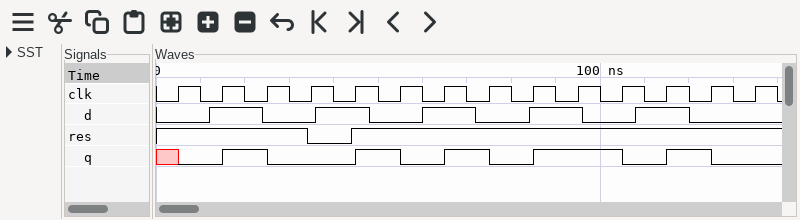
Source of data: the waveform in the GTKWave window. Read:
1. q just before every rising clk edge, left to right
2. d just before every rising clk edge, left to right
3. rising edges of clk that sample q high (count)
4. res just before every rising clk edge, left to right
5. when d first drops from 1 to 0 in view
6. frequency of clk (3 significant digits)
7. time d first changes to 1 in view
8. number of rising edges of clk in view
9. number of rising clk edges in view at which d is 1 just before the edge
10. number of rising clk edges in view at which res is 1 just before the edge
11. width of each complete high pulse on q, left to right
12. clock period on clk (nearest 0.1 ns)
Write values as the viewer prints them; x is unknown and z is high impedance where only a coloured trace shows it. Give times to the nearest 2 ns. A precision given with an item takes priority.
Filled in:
x 0 1 0 0 1 0 1 0 1 1 0 1 0
0 1 0 0 1 0 1 0 1 1 0 1 0 0
6
1 1 1 0 1 1 1 1 1 1 1 1 1 1
24 ns
100 MHz
12 ns
14
6
13
10 ns, 10 ns, 10 ns, 20 ns, 10 ns
10 ns
